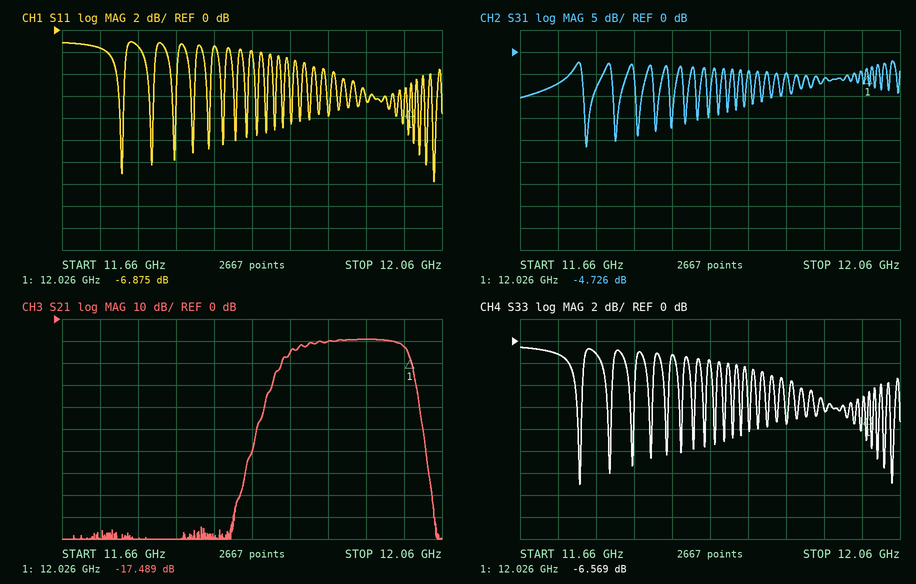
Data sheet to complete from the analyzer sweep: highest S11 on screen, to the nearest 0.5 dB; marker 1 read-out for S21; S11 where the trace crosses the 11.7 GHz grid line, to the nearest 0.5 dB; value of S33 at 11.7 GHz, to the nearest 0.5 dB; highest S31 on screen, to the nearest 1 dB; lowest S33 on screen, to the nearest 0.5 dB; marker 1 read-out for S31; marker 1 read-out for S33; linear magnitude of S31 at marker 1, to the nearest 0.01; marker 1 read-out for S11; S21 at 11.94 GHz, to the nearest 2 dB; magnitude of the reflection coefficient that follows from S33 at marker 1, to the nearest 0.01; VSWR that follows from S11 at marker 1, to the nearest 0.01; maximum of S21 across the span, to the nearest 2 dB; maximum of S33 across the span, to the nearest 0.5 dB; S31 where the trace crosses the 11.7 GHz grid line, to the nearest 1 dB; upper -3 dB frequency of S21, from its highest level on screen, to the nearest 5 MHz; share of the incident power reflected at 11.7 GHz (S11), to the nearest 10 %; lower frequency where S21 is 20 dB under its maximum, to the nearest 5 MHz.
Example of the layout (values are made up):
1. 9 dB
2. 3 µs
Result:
1. -1.0 dB
2. -17.489 dB
3. -1.5 dB
4. -1.0 dB
5. -2 dB
6. -13.0 dB
7. -4.726 dB
8. -6.569 dB
9. 0.58
10. -6.875 dB
11. -10 dB
12. 0.47
13. 2.66
14. -10 dB
15. -0.5 dB
16. -7 dB
17. 12.020 GHz
18. 70 %
19. 11.880 GHz
